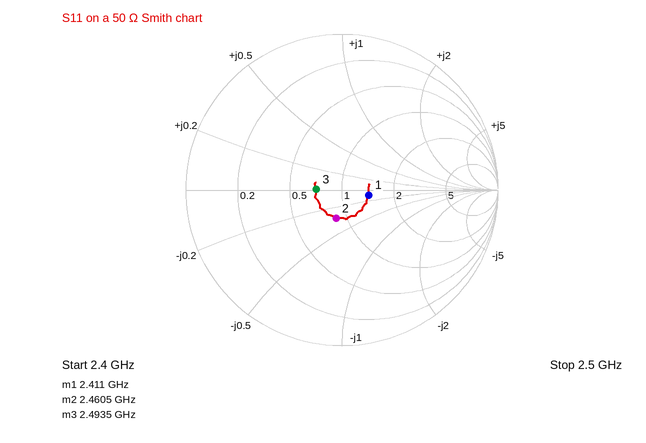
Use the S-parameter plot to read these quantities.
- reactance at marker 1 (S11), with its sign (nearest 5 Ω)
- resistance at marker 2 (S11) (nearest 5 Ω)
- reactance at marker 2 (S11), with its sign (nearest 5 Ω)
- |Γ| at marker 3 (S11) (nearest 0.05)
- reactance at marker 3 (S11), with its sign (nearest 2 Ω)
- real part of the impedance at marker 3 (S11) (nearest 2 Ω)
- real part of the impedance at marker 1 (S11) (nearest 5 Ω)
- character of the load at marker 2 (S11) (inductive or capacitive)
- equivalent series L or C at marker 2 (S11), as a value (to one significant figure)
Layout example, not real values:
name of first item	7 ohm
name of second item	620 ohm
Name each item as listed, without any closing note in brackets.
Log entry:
reactance at marker 1 (S11), with its sign	-5 Ω
resistance at marker 2 (S11)	45 Ω
reactance at marker 2 (S11), with its sign	-15 Ω
|Γ| at marker 3 (S11)	0.15
reactance at marker 3 (S11), with its sign	0 Ω
real part of the impedance at marker 3 (S11)	36 Ω
real part of the impedance at marker 1 (S11)	70 Ω
character of the load at marker 2 (S11)	capacitive
equivalent series L or C at marker 2 (S11), as a value	4 pF
